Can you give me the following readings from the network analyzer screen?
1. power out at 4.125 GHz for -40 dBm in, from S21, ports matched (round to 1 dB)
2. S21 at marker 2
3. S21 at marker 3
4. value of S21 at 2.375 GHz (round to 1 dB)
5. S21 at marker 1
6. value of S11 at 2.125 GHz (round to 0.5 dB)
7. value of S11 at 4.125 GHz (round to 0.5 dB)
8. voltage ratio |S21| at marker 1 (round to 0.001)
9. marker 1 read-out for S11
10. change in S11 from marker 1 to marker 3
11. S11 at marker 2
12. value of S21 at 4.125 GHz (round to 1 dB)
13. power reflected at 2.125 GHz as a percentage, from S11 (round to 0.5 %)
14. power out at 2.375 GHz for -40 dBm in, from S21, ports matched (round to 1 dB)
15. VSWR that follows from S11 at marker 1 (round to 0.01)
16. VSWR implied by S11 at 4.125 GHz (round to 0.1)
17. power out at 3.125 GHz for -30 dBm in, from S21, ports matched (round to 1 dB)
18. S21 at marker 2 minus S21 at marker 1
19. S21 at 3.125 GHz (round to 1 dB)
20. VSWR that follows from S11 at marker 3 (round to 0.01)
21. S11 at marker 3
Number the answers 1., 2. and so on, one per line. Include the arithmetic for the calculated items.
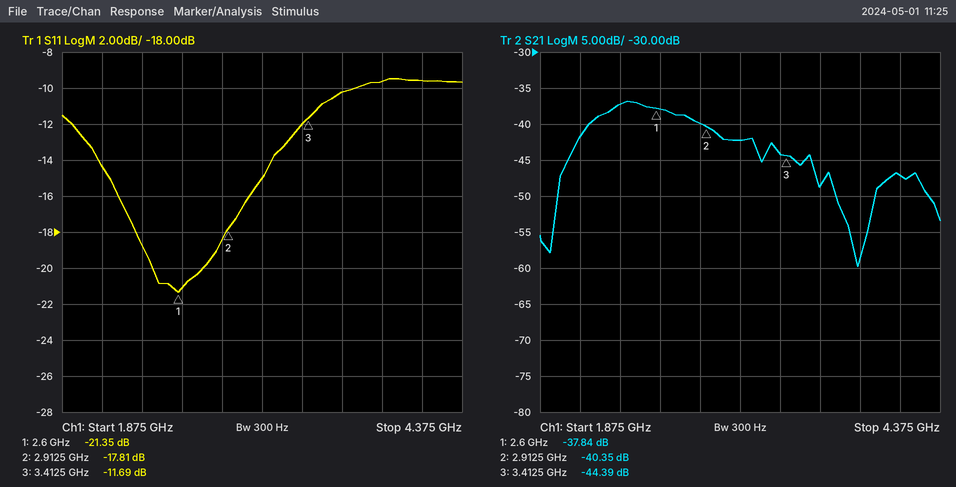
1. -40 dBm + (-47 dB) = -87 dBm
2. -40.35 dB
3. -44.39 dB
4. -37 dB
5. -37.84 dB
6. -14.5 dB
7. -9.5 dB
8. 10^(-37.84/20) ≈ 0.013
9. -21.35 dB
10. -11.69 − (-21.35) = 9.66 dB
11. -17.81 dB
12. -47 dB
13. 10^(-14.5/10) ≈ 3.5 %
14. -40 dBm + (-37 dB) = -77 dBm
15. (1 + 0.0856)/(1 − 0.0856) ≈ 1.19
16. |Γ| = 10^(-9.5/20) = 0.3350; VSWR = (1 + 0.3350)/(1 − 0.3350) ≈ 2.0
17. -30 dBm + (-42 dB) = -72 dBm
18. -40.35 − (-37.84) = -2.51 dB
19. -42 dB
20. (1 + 0.2603)/(1 − 0.2603) ≈ 1.70
21. -11.69 dB
